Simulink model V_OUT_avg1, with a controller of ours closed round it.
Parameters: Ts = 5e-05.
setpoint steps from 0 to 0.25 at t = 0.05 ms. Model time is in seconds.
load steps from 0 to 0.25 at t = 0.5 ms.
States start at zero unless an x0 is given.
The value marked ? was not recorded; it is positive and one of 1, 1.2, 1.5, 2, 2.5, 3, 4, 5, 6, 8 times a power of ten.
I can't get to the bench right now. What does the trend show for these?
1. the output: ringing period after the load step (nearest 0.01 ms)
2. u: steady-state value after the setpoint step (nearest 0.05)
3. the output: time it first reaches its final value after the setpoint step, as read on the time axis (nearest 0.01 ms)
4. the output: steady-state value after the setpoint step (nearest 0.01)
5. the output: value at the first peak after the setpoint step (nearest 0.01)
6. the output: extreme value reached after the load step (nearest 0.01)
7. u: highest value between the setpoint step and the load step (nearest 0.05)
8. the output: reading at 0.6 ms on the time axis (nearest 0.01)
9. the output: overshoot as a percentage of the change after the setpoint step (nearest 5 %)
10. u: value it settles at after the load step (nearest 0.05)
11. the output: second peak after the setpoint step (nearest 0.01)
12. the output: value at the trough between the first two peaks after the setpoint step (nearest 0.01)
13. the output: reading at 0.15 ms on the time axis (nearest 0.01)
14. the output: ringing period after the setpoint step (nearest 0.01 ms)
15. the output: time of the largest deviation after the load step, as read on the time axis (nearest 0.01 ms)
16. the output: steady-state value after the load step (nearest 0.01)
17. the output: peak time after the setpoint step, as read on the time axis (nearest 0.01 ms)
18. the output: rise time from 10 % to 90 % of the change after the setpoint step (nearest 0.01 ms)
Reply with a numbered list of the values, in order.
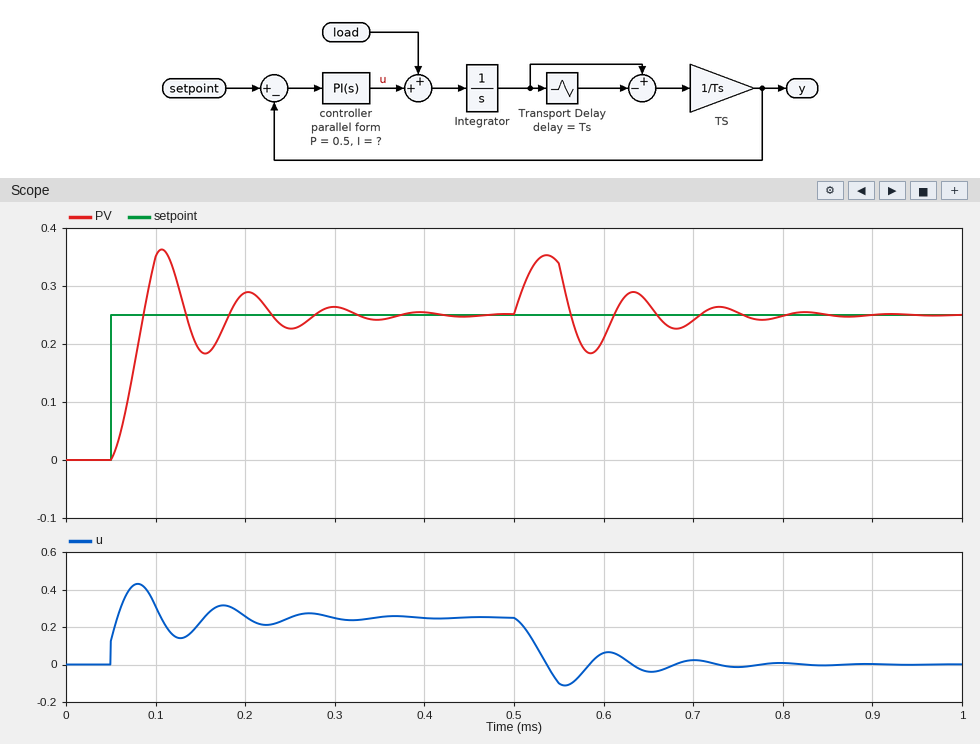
1. 0.10 ms
2. 0.25
3. 0.09 ms
4. 0.25
5. 0.36
6. 0.35
7. 0.45
8. 0.21
9. 45 %
10. 0.00
11. 0.29
12. 0.18
13. 0.19
14. 0.10 ms
15. 0.54 ms
16. 0.25
17. 0.11 ms
18. 0.03 ms
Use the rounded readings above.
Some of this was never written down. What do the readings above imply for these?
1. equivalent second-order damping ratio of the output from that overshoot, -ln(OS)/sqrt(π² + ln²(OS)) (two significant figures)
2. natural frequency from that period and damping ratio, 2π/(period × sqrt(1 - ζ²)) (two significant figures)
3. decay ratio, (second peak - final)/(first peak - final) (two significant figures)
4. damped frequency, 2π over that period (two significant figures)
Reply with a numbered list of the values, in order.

1. 0.25
2. 65 rad/ms
3. 0.36
4. 63 rad/ms
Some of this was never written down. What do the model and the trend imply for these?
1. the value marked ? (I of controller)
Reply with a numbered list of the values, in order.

1. 80000
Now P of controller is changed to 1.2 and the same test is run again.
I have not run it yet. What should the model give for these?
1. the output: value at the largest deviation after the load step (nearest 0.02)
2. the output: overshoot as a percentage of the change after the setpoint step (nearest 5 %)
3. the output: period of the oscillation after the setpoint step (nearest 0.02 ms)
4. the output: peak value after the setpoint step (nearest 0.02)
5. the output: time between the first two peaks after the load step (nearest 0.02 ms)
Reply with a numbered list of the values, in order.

1. 0.34
2. 35 %
3. 0.08 ms
4. 0.34
5. 0.08 ms
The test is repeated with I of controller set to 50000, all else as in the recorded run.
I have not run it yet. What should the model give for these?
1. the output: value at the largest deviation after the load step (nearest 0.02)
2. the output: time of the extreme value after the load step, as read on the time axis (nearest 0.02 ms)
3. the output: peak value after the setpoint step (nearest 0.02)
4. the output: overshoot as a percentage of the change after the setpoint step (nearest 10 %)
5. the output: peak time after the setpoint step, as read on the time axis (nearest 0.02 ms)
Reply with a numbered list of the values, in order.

1. 0.38
2. 0.54 ms
3. 0.30
4. 20 %
5. 0.12 ms
